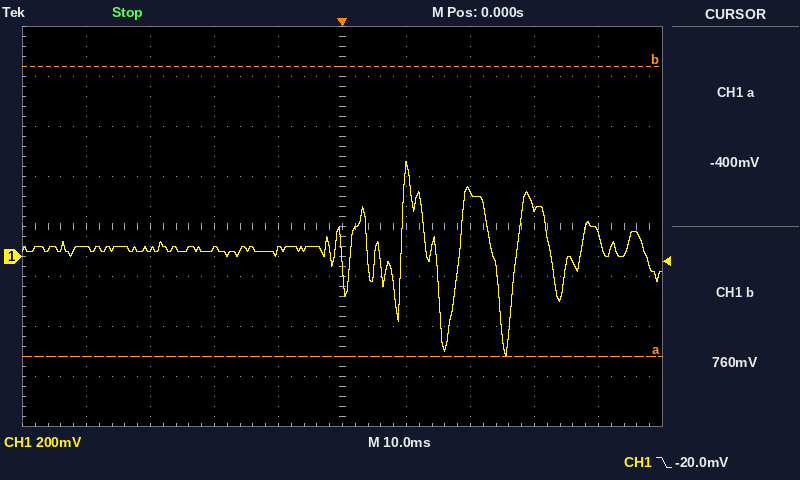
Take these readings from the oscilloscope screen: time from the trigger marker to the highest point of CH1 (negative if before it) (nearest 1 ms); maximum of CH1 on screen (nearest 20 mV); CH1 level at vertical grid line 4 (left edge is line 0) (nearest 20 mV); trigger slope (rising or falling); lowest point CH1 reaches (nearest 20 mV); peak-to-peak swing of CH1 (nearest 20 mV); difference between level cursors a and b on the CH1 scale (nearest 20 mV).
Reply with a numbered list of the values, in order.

1. +10 ms
2. 380 mV
3. 20 mV
4. falling
5. -400 mV
6. 780 mV
7. 1.16 V
